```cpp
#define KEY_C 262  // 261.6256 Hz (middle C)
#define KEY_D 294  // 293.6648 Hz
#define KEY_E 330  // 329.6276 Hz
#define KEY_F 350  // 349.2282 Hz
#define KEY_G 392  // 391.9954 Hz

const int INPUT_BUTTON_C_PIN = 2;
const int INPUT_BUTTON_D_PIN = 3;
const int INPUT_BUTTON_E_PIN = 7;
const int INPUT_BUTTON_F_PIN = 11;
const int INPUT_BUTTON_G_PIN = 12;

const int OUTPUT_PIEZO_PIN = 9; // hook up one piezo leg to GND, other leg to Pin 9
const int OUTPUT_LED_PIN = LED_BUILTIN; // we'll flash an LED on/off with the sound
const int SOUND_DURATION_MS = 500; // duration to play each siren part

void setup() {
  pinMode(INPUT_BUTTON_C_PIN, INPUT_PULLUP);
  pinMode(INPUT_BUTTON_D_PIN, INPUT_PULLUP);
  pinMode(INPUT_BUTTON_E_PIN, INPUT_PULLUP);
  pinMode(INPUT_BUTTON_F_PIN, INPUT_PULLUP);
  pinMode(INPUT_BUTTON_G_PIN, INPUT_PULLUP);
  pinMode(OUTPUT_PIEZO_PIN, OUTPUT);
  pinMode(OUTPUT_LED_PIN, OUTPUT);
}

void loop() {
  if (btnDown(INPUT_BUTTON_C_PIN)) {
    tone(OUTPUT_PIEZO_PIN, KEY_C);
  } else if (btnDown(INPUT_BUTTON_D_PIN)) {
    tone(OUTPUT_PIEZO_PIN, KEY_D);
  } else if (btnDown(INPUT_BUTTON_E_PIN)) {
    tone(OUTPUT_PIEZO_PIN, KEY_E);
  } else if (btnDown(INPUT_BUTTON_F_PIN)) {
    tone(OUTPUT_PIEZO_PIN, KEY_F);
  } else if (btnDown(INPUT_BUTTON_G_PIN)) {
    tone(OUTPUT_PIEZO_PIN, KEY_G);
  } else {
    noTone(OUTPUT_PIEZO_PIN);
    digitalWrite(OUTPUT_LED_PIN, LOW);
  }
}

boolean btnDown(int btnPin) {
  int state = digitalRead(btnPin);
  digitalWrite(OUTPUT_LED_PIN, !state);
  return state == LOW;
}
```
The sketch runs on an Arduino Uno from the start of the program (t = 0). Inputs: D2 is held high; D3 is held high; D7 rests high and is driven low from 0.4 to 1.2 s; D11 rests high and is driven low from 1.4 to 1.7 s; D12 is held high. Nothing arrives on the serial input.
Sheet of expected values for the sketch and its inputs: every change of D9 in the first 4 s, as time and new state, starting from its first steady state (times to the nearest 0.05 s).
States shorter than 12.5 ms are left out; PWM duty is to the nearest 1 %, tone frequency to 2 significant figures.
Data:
0 s low; 0.4 s tone 330 Hz; 1.2 s low; 1.4 s tone 350 Hz; 1.7 s low
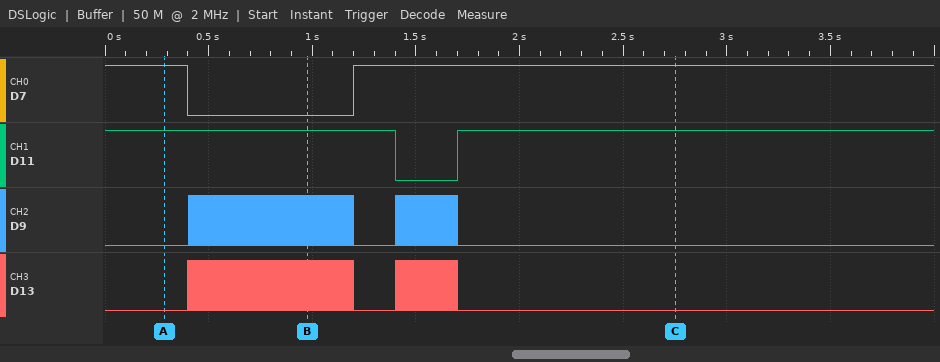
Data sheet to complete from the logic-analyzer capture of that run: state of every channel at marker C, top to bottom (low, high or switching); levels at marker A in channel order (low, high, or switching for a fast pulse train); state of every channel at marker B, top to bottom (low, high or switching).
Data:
D7 high, D11 high, D9 low, D13 low
D7 high, D11 high, D9 low, D13 low
D7 low, D11 high, D9 switching, D13 switching
